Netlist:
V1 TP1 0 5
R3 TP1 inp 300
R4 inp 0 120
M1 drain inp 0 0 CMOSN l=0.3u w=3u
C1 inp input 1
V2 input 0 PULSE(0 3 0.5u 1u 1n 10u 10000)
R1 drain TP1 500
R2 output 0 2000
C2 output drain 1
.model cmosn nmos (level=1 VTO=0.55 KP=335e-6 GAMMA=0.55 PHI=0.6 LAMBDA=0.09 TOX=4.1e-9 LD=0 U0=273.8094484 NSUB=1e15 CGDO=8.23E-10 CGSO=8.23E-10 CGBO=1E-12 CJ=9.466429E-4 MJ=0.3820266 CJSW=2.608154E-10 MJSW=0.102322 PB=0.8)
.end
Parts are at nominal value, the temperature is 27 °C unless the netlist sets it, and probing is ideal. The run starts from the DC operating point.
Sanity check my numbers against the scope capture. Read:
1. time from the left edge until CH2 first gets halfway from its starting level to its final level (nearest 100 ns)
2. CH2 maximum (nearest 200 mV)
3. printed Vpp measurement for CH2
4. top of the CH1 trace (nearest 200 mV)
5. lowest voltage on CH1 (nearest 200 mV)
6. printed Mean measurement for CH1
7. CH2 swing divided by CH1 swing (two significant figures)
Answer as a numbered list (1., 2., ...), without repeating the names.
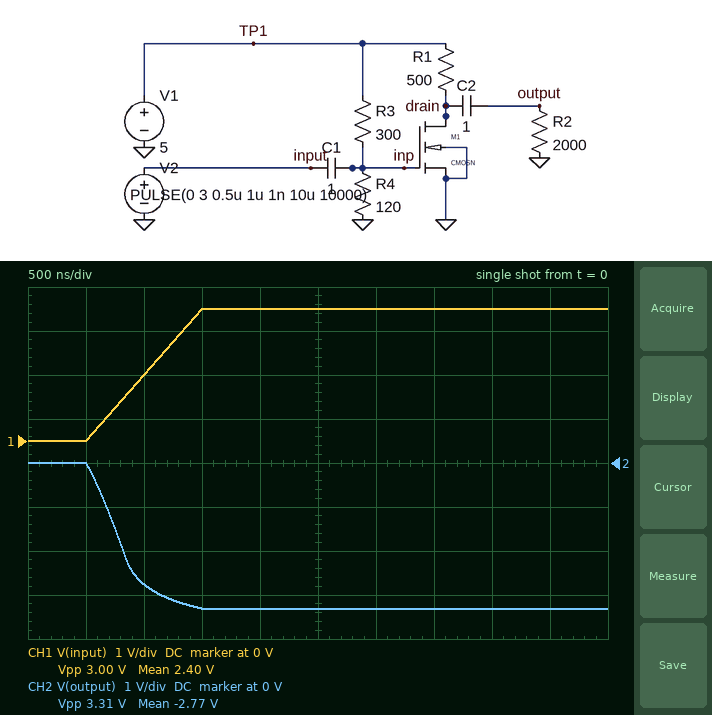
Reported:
1. 800 ns
2. 0 V
3. 3.31 V
4. 3.0 V
5. 0 V
6. 2.40 V
7. 1.1
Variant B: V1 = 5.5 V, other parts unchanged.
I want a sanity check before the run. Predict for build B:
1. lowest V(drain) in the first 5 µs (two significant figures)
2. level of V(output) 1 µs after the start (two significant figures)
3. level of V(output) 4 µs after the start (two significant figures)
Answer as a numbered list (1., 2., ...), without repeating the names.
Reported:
1. 850 mV
2. -2.9 V
3. -3.4 V
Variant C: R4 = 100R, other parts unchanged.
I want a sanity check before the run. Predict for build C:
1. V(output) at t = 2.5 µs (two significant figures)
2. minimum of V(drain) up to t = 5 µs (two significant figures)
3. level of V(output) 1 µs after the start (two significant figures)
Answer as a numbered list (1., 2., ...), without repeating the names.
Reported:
1. -3.6 V
2. 850 mV
3. -2.9 V
